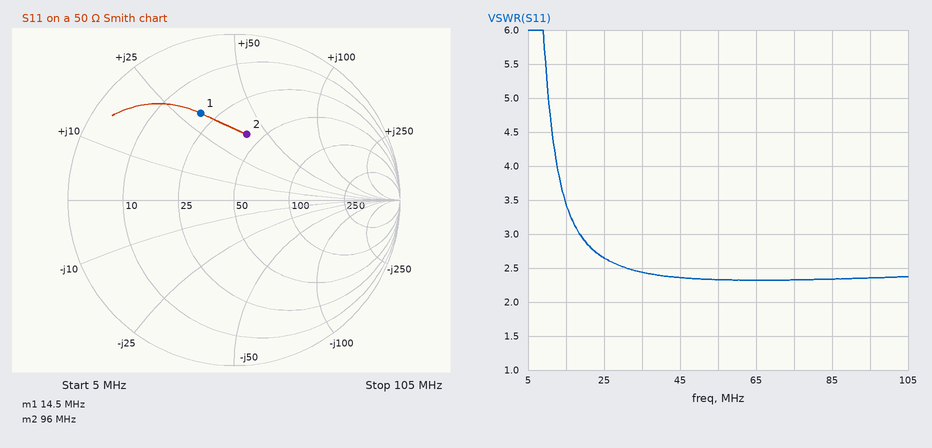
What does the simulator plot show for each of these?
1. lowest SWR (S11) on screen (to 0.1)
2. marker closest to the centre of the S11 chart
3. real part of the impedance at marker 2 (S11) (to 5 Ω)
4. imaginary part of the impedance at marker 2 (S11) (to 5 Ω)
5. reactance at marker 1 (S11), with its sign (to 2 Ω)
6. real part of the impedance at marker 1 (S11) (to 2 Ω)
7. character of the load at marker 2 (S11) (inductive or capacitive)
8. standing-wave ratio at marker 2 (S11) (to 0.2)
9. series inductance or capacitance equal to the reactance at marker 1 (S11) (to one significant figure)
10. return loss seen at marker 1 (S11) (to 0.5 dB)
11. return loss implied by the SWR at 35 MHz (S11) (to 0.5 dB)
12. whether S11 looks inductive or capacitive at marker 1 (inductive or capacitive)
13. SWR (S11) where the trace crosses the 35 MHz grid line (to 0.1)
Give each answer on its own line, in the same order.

2.3
marker 2
40 Ω
+40 Ω
+30 Ω
20 Ω
inductive
2.4
300 nH
5.0 dB
7.5 dB
inductive
2.4
